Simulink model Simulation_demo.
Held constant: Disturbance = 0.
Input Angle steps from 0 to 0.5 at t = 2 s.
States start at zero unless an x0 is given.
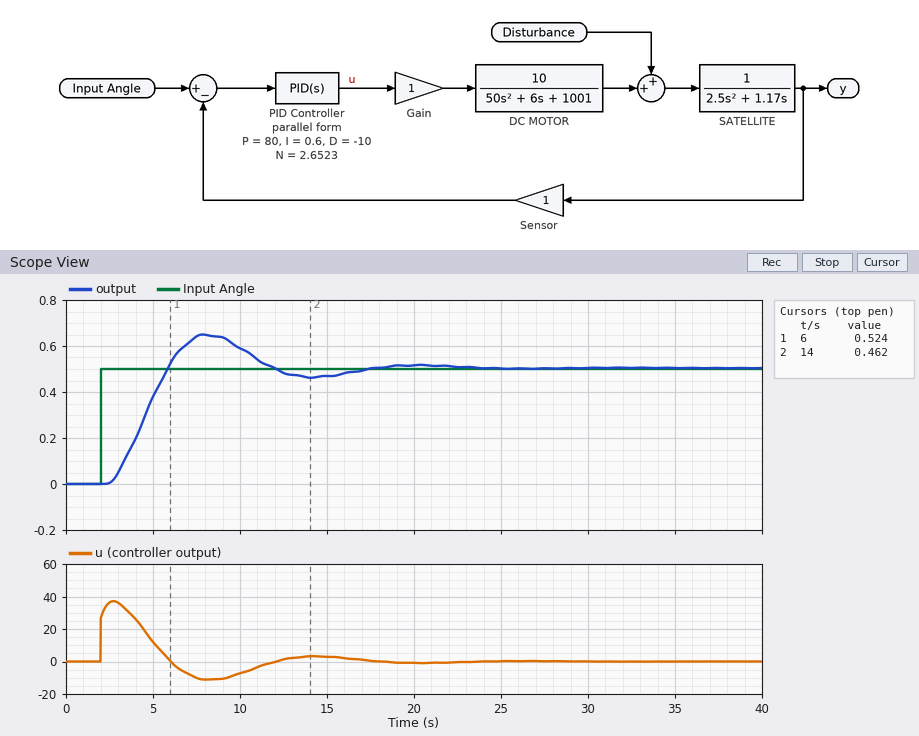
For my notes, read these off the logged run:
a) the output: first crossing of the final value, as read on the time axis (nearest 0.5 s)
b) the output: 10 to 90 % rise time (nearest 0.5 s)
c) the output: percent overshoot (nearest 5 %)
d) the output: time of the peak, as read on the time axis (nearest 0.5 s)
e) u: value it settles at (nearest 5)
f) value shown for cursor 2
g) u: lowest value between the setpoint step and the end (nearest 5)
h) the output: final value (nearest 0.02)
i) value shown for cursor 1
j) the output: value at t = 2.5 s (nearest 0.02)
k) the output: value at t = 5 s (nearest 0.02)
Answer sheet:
6.0 s
2.5 s
30 %
8.0 s
0
0.462
-10
0.50
0.524
0.00
0.38
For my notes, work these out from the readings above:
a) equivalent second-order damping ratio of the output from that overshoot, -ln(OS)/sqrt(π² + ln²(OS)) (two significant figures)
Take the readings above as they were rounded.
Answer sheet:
0.36
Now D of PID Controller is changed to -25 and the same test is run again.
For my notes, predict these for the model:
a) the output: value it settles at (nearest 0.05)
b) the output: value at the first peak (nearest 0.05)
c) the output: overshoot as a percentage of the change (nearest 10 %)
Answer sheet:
0.50
0.70
40 %
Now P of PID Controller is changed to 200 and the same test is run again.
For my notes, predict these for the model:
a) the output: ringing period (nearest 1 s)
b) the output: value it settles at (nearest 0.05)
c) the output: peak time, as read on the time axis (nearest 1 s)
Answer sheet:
7 s
0.50
6 s
